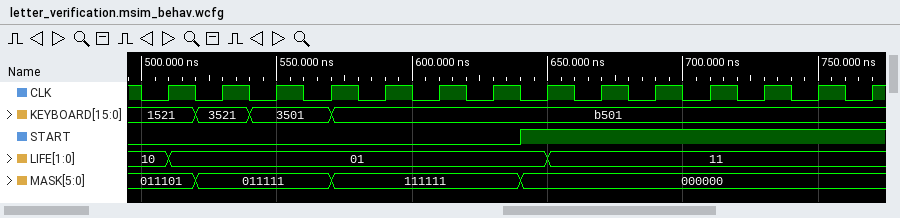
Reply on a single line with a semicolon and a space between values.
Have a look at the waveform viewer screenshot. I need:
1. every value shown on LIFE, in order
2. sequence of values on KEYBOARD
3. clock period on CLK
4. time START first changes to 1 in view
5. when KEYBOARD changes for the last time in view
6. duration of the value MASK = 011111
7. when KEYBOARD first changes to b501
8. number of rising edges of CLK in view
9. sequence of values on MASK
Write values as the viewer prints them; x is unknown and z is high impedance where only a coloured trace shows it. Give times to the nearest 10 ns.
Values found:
10, 01, 11; 1521, 3521, 3501, b501; 20 ns; 640 ns; 570 ns; 50 ns; 570 ns; 14; 011101, 011111, 111111, 000000
